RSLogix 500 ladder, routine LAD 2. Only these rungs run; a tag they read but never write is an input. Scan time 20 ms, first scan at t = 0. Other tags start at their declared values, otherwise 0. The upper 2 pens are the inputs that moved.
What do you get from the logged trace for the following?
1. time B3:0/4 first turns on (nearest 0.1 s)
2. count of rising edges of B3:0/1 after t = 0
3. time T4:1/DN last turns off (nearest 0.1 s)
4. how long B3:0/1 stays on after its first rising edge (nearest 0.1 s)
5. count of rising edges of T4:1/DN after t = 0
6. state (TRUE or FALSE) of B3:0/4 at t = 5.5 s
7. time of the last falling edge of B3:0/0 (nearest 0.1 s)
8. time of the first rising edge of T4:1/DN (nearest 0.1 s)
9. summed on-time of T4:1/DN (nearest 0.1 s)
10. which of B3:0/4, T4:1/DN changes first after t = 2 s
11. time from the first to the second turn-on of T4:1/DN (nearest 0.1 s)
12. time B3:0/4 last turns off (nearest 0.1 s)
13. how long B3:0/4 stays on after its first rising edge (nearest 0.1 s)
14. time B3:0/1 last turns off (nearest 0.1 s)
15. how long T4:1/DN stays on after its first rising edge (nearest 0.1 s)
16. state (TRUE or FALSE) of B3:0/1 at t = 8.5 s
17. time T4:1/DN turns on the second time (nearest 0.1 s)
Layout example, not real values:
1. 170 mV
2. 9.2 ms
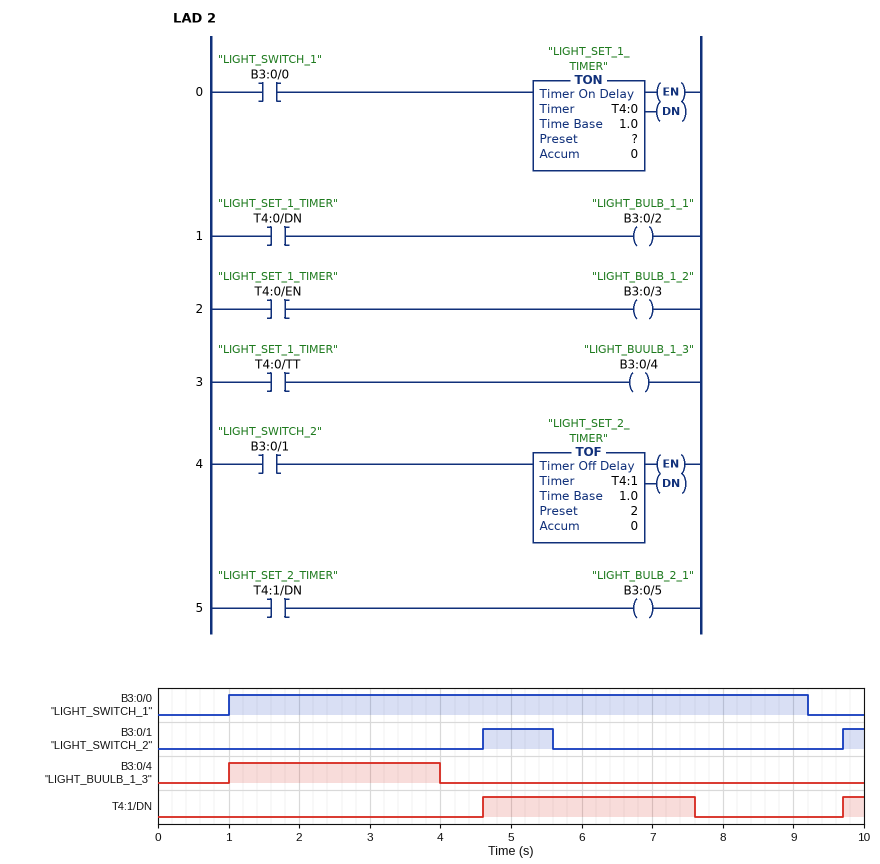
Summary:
1. 1.0 s
2. 2
3. 7.6 s
4. 1.0 s
5. 2
6. FALSE
7. 9.2 s
8. 4.6 s
9. 3.3 s
10. B3:0/4
11. 5.1 s
12. 4.0 s
13. 3.0 s
14. 5.6 s
15. 3.0 s
16. FALSE
17. 9.7 s
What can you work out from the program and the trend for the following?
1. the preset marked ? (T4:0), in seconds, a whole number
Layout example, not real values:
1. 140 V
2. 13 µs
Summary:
1. 3 s
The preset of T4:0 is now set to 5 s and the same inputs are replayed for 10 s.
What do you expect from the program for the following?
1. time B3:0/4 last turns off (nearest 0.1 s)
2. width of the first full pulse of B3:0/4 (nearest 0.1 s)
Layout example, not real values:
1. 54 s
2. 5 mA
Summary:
1. 6.0 s
2. 5.0 s
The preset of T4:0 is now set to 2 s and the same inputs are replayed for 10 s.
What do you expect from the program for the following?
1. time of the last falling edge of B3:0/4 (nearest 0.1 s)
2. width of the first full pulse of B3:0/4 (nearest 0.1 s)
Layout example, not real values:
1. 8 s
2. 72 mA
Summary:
1. 3.0 s
2. 2.0 s
